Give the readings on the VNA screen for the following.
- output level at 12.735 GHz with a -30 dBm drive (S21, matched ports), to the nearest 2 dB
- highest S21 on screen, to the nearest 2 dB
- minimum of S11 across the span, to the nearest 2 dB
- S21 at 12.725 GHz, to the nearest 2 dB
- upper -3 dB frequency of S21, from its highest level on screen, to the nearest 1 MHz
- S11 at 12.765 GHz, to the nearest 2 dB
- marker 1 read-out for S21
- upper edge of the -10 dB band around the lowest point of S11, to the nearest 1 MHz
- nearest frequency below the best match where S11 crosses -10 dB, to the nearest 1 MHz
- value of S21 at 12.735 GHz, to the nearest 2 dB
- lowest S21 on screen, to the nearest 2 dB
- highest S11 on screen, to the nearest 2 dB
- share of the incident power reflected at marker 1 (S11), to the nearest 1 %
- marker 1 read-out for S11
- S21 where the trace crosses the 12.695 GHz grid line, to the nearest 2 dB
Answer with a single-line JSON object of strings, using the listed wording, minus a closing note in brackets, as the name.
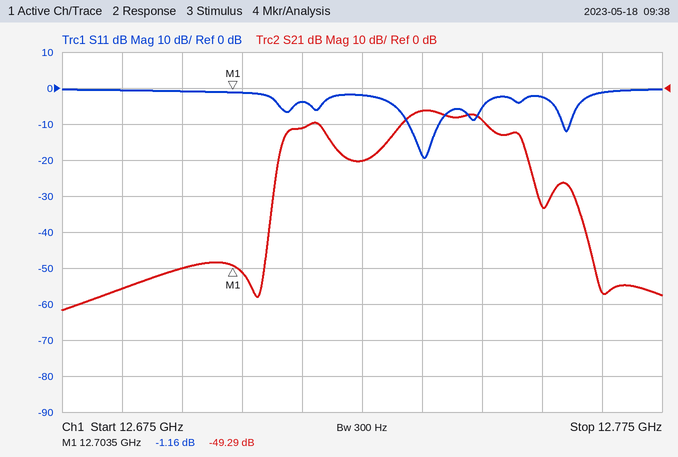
{"output level at 12.735 GHz with a -30 dBm drive (S21, matched ports), to the nearest 2 dB": "-36 dBm", "highest S21 on screen, to the nearest 2 dB": "-6 dB", "minimum of S11 across the span, to the nearest 2 dB": "-20 dB", "S21 at 12.725 GHz, to the nearest 2 dB": "-20 dB", "upper -3 dB frequency of S21, from its highest level on screen, to the nearest 1 MHz": "12.745 GHz", "S11 at 12.765 GHz, to the nearest 2 dB": "-2 dB", "marker 1 read-out for S21": "-49.29 dB", "upper edge of the -10 dB band around the lowest point of S11, to the nearest 1 MHz": "12.738 GHz", "nearest frequency below the best match where S11 crosses -10 dB, to the nearest 1 MHz": "12.733 GHz", "value of S21 at 12.735 GHz, to the nearest 2 dB": "-6 dB", "lowest S21 on screen, to the nearest 2 dB": "-62 dB", "highest S11 on screen, to the nearest 2 dB": "0 dB", "share of the incident power reflected at marker 1 (S11), to the nearest 1 %": "77 %", "marker 1 read-out for S11": "-1.16 dB", "S21 where the trace crosses the 12.695 GHz grid line, to the nearest 2 dB": "-50 dB"}
